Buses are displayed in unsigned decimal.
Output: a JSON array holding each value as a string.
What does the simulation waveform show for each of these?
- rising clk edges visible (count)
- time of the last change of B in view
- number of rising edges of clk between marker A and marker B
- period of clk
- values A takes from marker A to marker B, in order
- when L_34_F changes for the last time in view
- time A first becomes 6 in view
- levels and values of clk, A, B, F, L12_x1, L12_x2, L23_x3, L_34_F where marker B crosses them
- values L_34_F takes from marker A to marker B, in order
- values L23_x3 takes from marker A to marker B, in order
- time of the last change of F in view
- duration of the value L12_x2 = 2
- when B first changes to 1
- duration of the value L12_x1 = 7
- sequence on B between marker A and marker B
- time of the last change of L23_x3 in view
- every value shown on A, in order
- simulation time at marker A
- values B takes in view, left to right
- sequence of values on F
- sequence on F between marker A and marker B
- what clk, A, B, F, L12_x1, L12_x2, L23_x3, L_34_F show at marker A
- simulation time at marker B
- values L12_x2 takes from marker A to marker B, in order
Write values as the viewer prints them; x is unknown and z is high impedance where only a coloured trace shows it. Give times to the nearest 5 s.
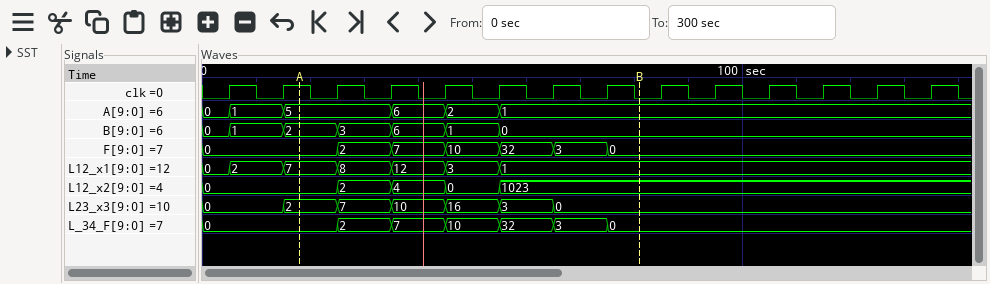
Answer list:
["14", "55 s", "6", "10 s", "5, 6, 2, 1", "75 s", "35 s", "clk=0, A=1, B=0, F=0, L12_x1=1, L12_x2=1023, L23_x3=0, L_34_F=0", "0, 2, 7, 10, 32, 3, 0", "2, 7, 10, 16, 3, 0", "75 s", "10 s", "5 s", "10 s", "2, 3, 6, 1, 0", "65 s", "0, 1, 5, 6, 2, 1", "20 s", "0, 1, 2, 3, 6, 1, 0", "0, 2, 7, 10, 32, 3, 0", "0, 2, 7, 10, 32, 3, 0", "clk=1, A=5, B=2, F=0, L12_x1=7, L12_x2=0, L23_x3=2, L_34_F=0", "80 s", "0, 2, 4, 0, 1023"]
